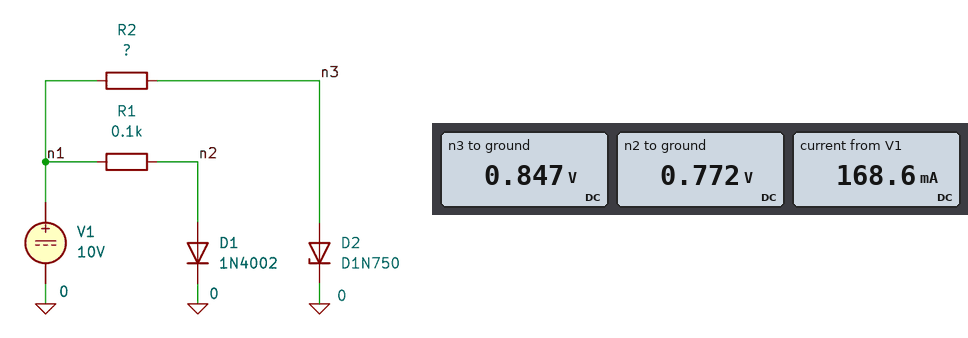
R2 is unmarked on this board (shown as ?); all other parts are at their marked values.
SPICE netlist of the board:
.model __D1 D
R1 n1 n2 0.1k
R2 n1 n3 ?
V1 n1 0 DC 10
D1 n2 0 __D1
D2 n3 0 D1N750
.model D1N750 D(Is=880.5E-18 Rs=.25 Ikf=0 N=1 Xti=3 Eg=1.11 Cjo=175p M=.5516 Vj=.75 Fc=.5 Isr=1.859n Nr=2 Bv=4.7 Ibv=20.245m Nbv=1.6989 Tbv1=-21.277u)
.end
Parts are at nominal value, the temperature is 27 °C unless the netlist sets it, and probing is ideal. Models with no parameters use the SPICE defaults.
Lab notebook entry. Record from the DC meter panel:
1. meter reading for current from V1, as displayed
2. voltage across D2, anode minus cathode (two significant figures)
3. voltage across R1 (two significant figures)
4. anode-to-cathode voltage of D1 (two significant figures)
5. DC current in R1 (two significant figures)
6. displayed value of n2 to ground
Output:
168.6 mA
850 mV
9.2 V
770 mV
92 mA
0.772 V
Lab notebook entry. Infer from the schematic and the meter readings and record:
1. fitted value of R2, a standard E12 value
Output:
120 Ω
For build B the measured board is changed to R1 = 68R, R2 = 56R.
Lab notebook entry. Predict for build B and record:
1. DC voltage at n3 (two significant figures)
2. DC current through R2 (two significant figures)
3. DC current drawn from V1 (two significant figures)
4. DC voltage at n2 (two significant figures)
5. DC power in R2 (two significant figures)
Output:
890 mV
160 mA
300 mA
780 mV
1.5 W
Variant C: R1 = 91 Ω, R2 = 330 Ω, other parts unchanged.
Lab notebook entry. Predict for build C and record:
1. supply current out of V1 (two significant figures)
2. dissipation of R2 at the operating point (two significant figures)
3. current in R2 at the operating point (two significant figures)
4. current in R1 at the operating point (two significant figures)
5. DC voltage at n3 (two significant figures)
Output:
130 mA
260 mW
28 mA
100 mA
810 mV
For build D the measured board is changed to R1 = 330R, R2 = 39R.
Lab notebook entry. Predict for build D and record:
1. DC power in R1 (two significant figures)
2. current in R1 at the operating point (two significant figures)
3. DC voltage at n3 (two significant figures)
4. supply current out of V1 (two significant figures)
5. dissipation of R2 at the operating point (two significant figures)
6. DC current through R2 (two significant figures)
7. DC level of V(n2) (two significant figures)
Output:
260 mW
28 mA
920 mV
260 mA
2.1 W
230 mA
740 mV
